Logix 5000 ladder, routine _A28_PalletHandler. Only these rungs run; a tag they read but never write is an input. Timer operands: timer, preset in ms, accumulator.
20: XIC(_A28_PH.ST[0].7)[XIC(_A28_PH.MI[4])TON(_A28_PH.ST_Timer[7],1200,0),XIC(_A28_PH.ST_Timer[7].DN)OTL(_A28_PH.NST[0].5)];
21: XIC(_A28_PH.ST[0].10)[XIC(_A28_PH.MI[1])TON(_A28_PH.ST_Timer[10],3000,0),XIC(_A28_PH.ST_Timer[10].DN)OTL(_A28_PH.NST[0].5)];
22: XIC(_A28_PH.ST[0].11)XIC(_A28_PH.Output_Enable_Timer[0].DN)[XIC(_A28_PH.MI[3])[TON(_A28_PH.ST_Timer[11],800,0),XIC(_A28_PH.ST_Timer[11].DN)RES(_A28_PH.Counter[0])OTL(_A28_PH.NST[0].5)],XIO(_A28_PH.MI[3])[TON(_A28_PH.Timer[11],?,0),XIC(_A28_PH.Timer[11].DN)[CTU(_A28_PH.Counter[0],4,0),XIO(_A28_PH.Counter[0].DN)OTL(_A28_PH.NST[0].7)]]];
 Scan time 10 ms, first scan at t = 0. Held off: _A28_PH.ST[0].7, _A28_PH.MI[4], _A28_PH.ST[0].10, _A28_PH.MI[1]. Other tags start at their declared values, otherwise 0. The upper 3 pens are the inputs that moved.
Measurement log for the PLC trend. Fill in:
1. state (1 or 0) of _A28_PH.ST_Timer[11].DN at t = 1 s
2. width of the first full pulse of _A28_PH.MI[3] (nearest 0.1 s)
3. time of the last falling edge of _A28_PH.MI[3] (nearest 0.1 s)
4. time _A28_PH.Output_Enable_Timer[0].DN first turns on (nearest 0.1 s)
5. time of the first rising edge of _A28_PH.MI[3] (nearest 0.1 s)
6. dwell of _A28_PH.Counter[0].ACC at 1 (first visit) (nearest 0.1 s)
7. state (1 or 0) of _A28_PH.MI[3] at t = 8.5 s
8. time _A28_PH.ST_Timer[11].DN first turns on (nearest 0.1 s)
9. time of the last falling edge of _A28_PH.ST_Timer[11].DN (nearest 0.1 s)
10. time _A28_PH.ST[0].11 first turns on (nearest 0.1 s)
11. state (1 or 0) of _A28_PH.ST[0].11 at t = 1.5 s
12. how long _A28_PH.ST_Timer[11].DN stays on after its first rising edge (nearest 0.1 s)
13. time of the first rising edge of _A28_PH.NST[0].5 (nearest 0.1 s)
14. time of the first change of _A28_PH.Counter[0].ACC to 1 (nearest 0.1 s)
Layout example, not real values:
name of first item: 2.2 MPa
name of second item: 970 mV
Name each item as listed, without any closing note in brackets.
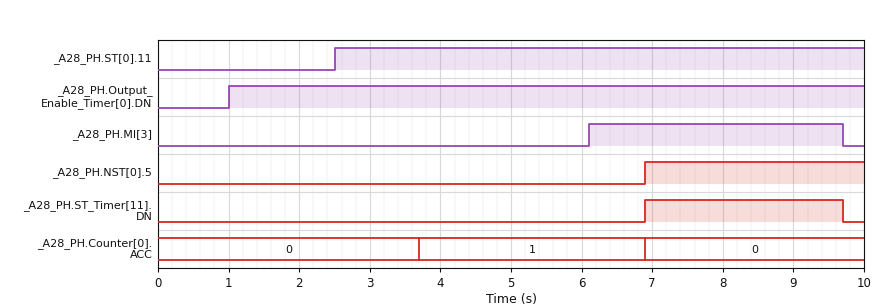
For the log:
state (1 or 0) of _A28_PH.ST_Timer[11].DN at t = 1 s: 0
width of the first full pulse of _A28_PH.MI[3]: 3.6 s
time of the last falling edge of _A28_PH.MI[3]: 9.7 s
time _A28_PH.Output_Enable_Timer[0].DN first turns on: 1.0 s
time of the first rising edge of _A28_PH.MI[3]: 6.1 s
dwell of _A28_PH.Counter[0].ACC at 1 (first visit): 3.2 s
state (1 or 0) of _A28_PH.MI[3] at t = 8.5 s: 1
time _A28_PH.ST_Timer[11].DN first turns on: 6.9 s
time of the last falling edge of _A28_PH.ST_Timer[11].DN: 9.7 s
time _A28_PH.ST[0].11 first turns on: 2.5 s
state (1 or 0) of _A28_PH.ST[0].11 at t = 1.5 s: 0
how long _A28_PH.ST_Timer[11].DN stays on after its first rising edge: 2.8 s
time of the first rising edge of _A28_PH.NST[0].5: 6.9 s
time of the first change of _A28_PH.Counter[0].ACC to 1: 3.7 s
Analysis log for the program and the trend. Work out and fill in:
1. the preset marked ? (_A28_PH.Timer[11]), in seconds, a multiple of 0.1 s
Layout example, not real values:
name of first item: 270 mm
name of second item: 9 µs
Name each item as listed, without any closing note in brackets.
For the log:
the preset marked ? (_A28_PH.Timer[11]), in seconds, a multiple of 0.1 s: 1.2 s
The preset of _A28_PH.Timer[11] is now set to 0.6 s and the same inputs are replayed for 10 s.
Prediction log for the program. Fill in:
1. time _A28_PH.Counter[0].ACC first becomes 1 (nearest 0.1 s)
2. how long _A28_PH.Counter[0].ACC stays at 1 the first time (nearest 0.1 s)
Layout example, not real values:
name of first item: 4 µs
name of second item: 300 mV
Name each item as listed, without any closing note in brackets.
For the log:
time _A28_PH.Counter[0].ACC first becomes 1: 3.1 s
how long _A28_PH.Counter[0].ACC stays at 1 the first time: 3.8 s
